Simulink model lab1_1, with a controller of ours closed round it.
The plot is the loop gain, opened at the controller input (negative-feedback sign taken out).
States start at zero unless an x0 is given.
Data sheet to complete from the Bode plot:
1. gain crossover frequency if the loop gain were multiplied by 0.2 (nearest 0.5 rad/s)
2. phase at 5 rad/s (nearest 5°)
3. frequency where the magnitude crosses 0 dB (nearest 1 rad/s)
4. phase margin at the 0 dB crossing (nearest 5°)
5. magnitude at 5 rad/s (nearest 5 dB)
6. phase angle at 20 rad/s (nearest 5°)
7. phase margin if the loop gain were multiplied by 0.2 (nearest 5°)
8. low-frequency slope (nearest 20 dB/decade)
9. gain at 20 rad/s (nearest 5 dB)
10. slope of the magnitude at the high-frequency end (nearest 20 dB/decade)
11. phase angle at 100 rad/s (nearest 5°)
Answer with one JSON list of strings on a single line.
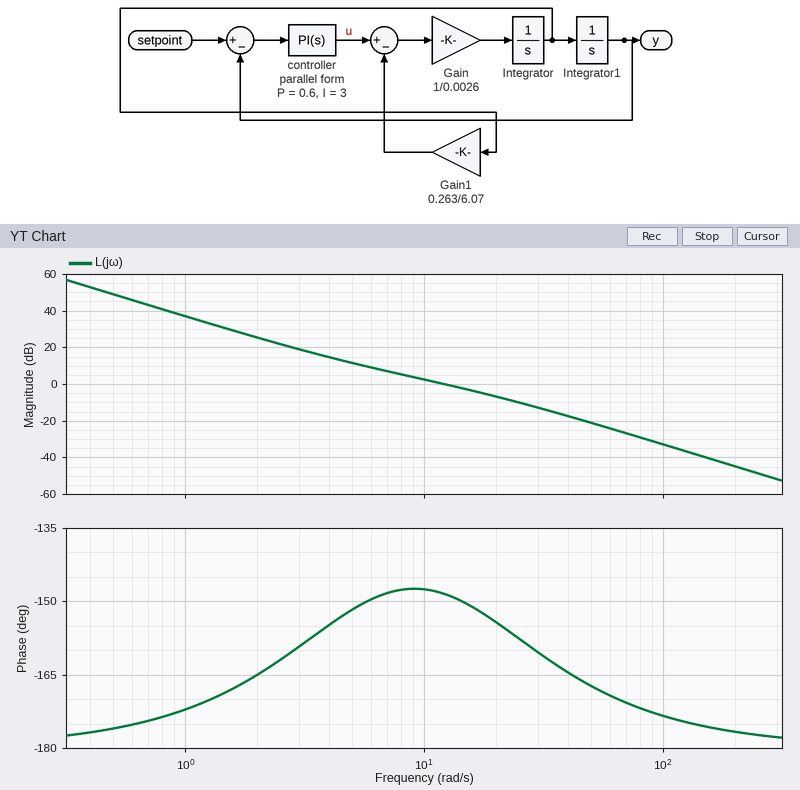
["4.0 rad/s", "-150°", "12 rad/s", "30°", "10 dB", "-155°", "25°", "-40 dB/decade", "-5 dB", "-40 dB/decade", "-175°"]
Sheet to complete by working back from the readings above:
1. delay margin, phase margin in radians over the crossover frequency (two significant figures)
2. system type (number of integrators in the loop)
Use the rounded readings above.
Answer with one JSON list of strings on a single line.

["0.044 s", "2"]
